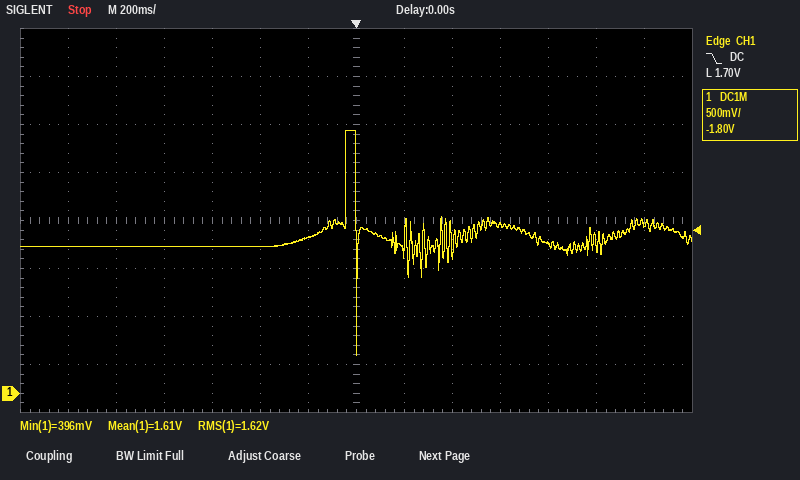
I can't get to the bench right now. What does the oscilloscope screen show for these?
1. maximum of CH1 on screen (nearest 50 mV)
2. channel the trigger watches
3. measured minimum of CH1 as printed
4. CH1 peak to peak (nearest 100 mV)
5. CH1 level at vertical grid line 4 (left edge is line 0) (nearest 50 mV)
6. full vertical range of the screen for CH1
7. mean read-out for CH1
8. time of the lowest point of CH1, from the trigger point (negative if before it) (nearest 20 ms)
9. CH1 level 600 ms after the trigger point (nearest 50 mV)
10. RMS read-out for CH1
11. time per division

2.75 V
CH1
396 mV
2.30 V
1.55 V
4 V
1.61 V
0 ms
1.75 V
1.62 V
200 ms
